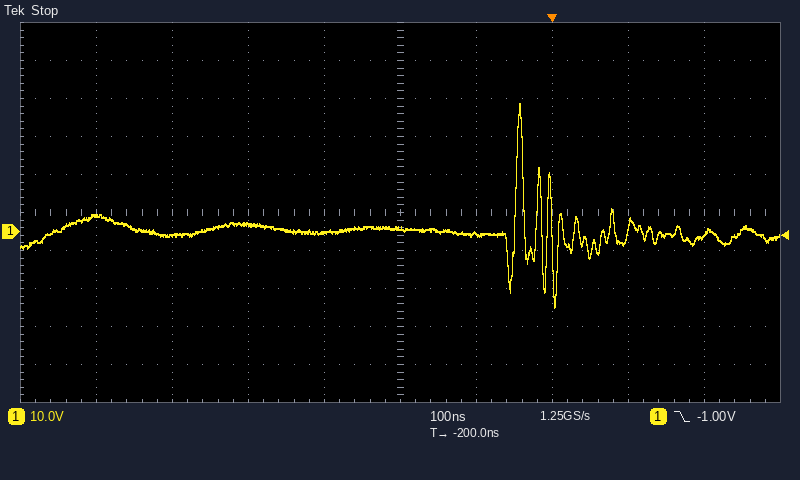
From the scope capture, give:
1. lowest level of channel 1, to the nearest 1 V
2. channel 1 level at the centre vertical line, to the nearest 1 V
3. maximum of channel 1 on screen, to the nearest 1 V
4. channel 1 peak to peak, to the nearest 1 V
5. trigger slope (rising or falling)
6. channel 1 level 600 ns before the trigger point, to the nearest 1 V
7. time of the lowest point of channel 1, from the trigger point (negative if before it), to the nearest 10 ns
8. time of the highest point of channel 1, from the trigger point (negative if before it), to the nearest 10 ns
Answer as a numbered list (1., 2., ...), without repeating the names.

1. -20 V
2. 1 V
3. 34 V
4. 54 V
5. falling
6. 4 V
7. 0 ns
8. -40 ns
